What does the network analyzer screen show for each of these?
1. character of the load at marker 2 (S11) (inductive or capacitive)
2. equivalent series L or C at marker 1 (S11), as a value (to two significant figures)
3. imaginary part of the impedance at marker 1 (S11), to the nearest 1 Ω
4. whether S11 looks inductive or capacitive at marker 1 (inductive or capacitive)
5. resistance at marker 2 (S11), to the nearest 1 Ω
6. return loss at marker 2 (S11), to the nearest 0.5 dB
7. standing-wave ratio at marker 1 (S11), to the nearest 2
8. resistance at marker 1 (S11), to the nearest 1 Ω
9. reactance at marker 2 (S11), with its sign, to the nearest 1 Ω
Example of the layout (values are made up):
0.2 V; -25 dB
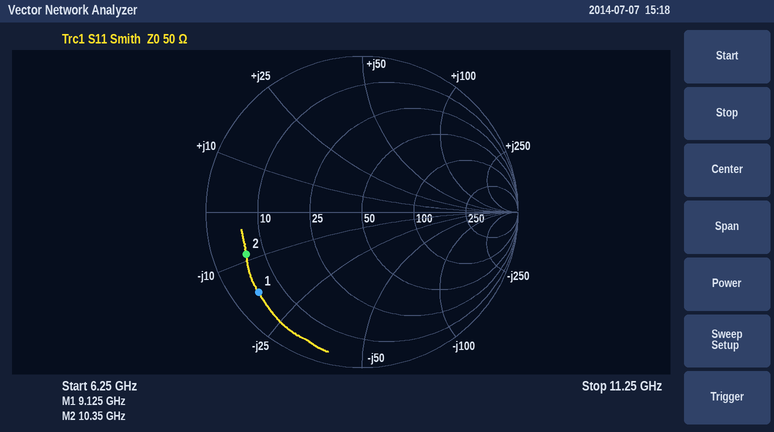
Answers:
capacitive; 1.0 pF; -17 Ω; capacitive; 6 Ω; 2.0 dB; 12; 5 Ω; -9 Ω
